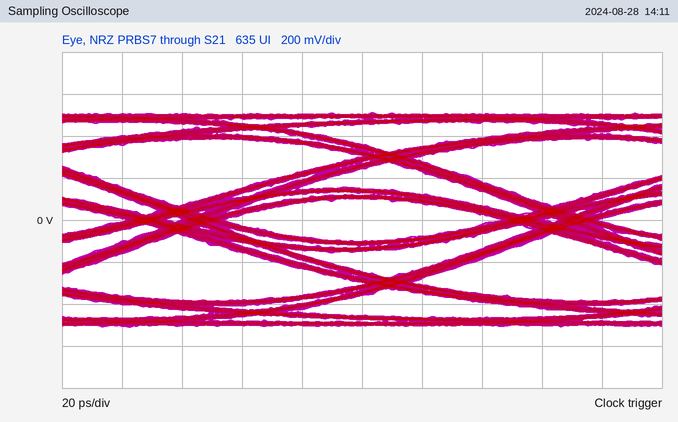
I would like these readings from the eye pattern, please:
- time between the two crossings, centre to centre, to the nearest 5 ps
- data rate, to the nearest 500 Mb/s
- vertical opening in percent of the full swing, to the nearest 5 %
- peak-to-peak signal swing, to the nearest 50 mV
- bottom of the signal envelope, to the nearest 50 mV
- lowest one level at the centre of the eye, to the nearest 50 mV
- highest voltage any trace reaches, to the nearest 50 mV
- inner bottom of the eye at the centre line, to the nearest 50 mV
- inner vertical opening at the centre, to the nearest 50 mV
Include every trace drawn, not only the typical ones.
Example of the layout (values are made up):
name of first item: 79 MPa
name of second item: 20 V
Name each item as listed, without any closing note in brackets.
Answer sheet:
time between the two crossings, centre to centre, to the nearest 5 ps: 125 ps
data rate, to the nearest 500 Mb/s: 8.0 Gb/s
vertical opening in percent of the full swing, to the nearest 5 %: 20 %
peak-to-peak signal swing, to the nearest 50 mV: 1.00 V
bottom of the signal envelope, to the nearest 50 mV: -500 mV
lowest one level at the centre of the eye, to the nearest 50 mV: 100 mV
highest voltage any trace reaches, to the nearest 50 mV: 500 mV
inner bottom of the eye at the centre line, to the nearest 50 mV: -100 mV
inner vertical opening at the centre, to the nearest 50 mV: 200 mV
